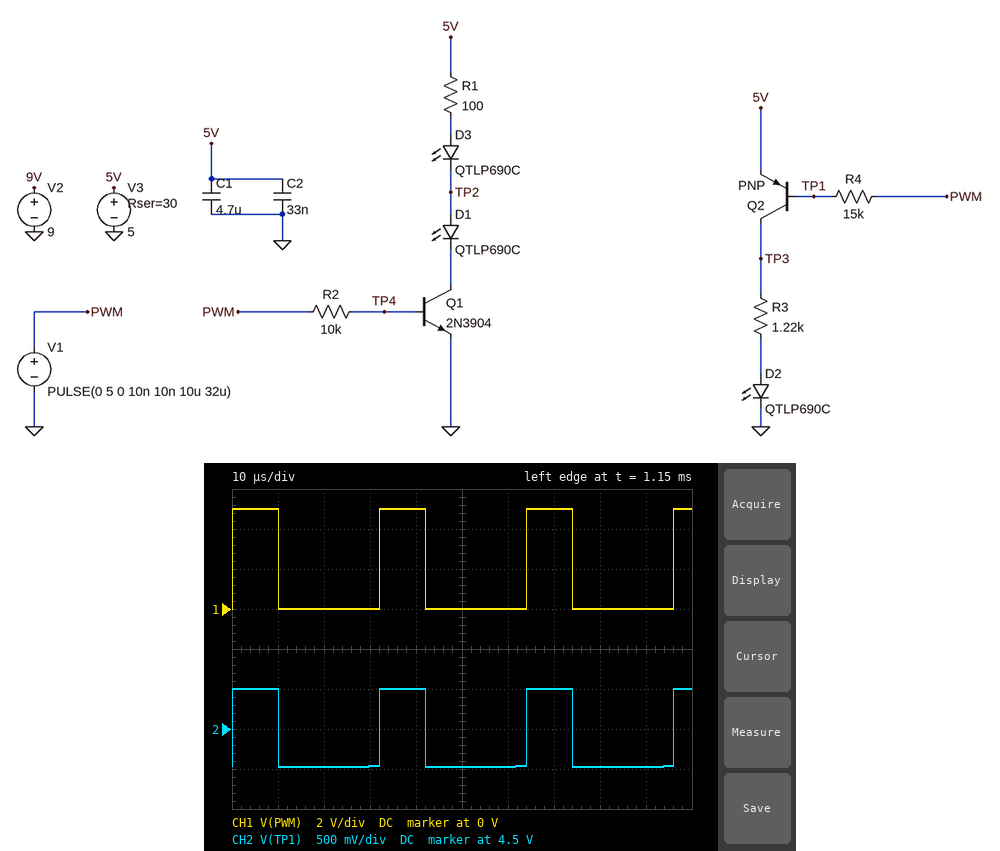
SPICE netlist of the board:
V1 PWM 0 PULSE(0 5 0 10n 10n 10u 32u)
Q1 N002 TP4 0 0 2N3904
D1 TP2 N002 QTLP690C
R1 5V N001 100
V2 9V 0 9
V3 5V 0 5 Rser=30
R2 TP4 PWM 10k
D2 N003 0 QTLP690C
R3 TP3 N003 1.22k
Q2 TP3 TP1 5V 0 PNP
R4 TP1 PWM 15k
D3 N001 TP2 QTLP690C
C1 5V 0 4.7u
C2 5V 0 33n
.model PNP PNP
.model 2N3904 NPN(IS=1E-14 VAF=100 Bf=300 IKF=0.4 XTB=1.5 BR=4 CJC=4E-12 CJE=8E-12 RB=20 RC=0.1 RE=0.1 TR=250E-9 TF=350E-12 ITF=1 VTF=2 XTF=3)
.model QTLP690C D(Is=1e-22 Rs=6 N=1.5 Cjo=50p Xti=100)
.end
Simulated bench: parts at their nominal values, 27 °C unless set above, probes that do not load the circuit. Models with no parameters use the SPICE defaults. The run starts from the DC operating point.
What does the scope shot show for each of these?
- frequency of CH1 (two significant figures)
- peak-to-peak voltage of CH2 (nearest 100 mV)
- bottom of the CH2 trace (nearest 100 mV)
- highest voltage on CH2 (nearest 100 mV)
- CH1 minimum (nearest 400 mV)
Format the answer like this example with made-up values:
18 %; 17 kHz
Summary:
31 kHz; 1.0 V; 4.0 V; 5.0 V; 0 V
